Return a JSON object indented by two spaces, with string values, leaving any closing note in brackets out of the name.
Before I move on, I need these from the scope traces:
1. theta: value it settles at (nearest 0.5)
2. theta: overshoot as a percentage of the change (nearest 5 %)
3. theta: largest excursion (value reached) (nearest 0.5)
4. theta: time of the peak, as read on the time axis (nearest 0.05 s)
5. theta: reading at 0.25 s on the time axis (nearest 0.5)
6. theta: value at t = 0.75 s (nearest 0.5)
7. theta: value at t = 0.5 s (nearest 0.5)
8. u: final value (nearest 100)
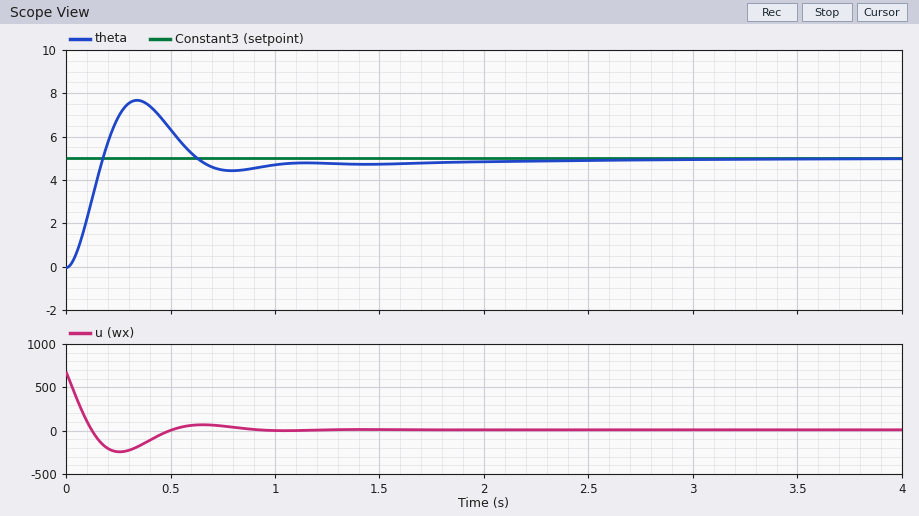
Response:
{
  "theta: value it settles at": "5.0",
  "theta: overshoot as a percentage of the change": "55 %",
  "theta: largest excursion (value reached)": "7.5",
  "theta: time of the peak, as read on the time axis": "0.35 s",
  "theta: reading at 0.25 s on the time axis": "7.0",
  "theta: value at t = 0.75 s": "4.5",
  "theta: value at t = 0.5 s": "6.5",
  "u: final value": "0"
}
